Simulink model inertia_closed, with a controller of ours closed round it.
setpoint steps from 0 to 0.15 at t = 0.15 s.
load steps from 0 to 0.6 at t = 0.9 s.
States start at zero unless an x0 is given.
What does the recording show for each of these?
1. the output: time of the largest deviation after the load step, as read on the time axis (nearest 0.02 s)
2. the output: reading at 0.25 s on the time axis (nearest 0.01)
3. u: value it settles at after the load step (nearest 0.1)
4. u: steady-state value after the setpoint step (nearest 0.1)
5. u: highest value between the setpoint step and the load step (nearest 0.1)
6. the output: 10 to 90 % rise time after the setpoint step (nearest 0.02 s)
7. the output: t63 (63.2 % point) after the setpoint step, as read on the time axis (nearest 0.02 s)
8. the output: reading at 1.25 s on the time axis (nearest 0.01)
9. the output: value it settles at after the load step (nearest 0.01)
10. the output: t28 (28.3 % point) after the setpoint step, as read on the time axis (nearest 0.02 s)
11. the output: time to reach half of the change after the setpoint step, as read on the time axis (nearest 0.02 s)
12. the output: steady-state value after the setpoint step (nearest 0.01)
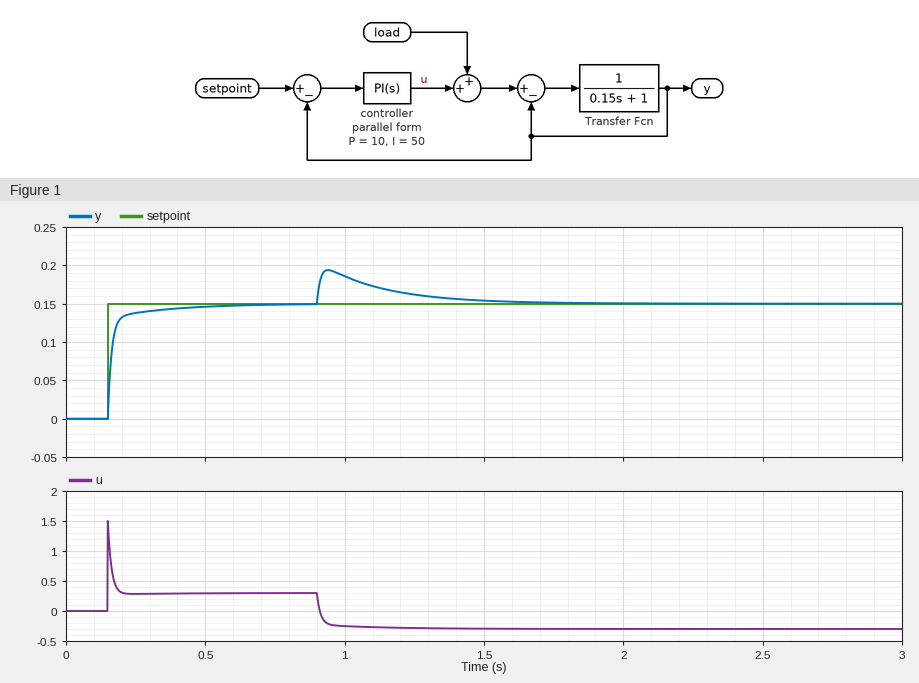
0.94 s
0.14
-0.3
0.3
1.5
0.06 s
0.16 s
0.16
0.15
0.16 s
0.16 s
0.15
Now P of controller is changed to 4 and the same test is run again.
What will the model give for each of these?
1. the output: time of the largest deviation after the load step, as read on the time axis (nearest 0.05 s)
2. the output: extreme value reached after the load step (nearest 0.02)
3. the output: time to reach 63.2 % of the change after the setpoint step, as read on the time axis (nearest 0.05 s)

0.95 s
0.22
0.20 s
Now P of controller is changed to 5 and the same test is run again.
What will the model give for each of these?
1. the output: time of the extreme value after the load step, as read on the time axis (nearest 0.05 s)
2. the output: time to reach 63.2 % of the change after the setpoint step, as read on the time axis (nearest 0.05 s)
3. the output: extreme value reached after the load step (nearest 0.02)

0.95 s
0.20 s
0.22
